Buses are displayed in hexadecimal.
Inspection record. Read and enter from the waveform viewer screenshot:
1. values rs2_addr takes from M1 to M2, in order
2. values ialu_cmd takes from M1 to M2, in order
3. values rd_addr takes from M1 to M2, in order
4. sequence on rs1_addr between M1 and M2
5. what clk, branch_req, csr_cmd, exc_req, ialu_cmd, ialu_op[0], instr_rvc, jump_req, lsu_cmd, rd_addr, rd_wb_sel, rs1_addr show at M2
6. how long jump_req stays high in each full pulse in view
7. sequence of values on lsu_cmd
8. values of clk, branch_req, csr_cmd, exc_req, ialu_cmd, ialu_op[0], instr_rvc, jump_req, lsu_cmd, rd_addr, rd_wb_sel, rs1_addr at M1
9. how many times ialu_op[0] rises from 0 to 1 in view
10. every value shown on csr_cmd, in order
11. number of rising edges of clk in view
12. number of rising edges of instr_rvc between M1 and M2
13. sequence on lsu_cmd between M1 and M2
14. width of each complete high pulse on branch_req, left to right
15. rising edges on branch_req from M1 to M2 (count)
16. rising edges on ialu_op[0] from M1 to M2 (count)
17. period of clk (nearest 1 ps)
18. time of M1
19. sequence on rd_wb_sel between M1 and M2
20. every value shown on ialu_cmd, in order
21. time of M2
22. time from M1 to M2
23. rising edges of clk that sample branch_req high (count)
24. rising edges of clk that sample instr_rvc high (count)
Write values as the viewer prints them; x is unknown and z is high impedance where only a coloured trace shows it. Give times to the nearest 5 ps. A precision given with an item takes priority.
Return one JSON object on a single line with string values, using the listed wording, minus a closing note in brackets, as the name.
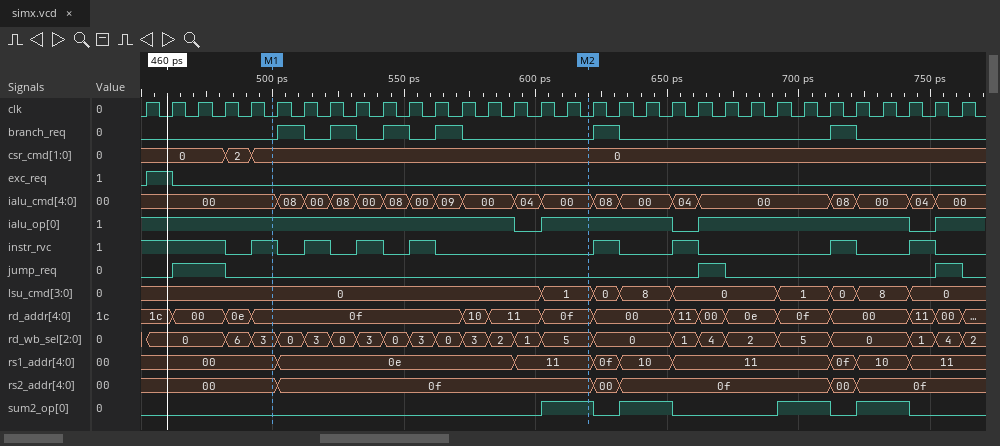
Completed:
{"values rs2_addr takes from M1 to M2, in order": "00, 0f", "values ialu_cmd takes from M1 to M2, in order": "00, 08, 00, 08, 00, 08, 00, 09, 00, 04, 00", "values rd_addr takes from M1 to M2, in order": "0f, 10, 11, 0f", "sequence on rs1_addr between M1 and M2": "00, 0e, 11", "what clk, branch_req, csr_cmd, exc_req, ialu_cmd, ialu_op[0], instr_rvc, jump_req, lsu_cmd, rd_addr, rd_wb_sel, rs1_addr show at M2": "clk=0, branch_req=0, csr_cmd=0, exc_req=0, ialu_cmd=00, ialu_op[0]=1, instr_rvc=0, jump_req=0, lsu_cmd=1, rd_addr=0f, rd_wb_sel=5, rs1_addr=11", "how long jump_req stays high in each full pulse in view": "20 ps, 10 ps, 10 ps", "sequence of values on lsu_cmd": "0, 1, 0, 8, 0, 1, 0, 8, 0", "values of clk, branch_req, csr_cmd, exc_req, ialu_cmd, ialu_op[0], instr_rvc, jump_req, lsu_cmd, rd_addr, rd_wb_sel, rs1_addr at M1": "clk=0, branch_req=0, csr_cmd=0, exc_req=0, ialu_cmd=00, ialu_op[0]=1, instr_rvc=1, jump_req=0, lsu_cmd=0, rd_addr=0f, rd_wb_sel=3, rs1_addr=00", "how many times ialu_op[0] rises from 0 to 1 in view": "3", "every value shown on csr_cmd, in order": "0, 2, 0", "number of rising edges of clk in view": "32", "number of rising edges of instr_rvc between M1 and M2": "3", "sequence on lsu_cmd between M1 and M2": "0, 1", "width of each complete high pulse on branch_req, left to right": "10 ps, 10 ps, 10 ps, 10 ps, 10 ps, 10 ps", "rising edges on branch_req from M1 to M2": "4", "rising edges on ialu_op[0] from M1 to M2": "1", "period of clk": "10 ps", "time of M1": "500 ps", "sequence on rd_wb_sel between M1 and M2": "3, 0, 3, 0, 3, 0, 3, 0, 3, 2, 1, 5", "every value shown on ialu_cmd, in order": "00, 08, 00, 08, 00, 08, 00, 09, 00, 04, 00, 08, 00, 04, 00, 08, 00, 04, 00", "time of M2": "620 ps", "time from M1 to M2": "120 ps", "rising edges of clk that sample branch_req high": "6", "rising edges of clk that sample instr_rvc high": "12"}
